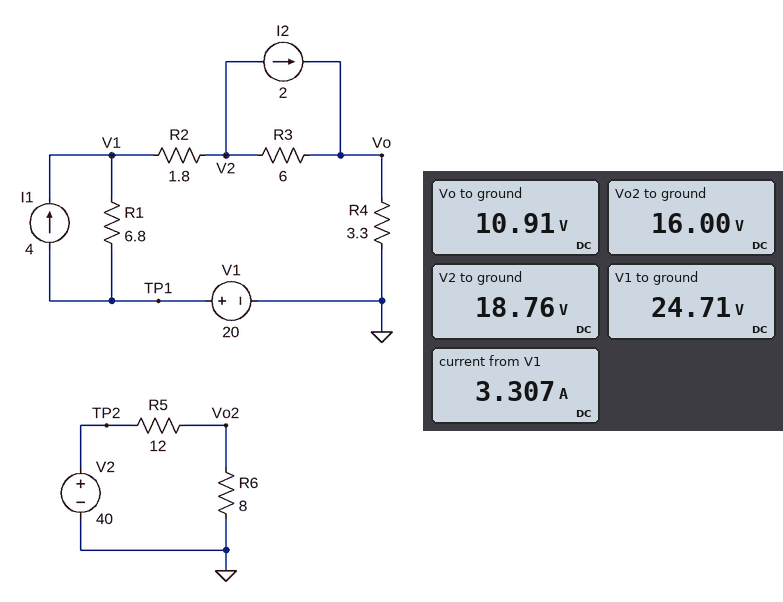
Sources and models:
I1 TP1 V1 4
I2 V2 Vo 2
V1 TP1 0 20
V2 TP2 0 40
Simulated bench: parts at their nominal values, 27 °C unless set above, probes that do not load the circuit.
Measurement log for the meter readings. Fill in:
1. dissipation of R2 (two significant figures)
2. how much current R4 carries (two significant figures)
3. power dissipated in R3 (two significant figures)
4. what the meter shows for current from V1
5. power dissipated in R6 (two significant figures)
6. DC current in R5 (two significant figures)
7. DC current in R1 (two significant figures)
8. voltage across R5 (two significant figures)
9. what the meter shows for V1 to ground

20 W
3.3 A
10 W
3.307 A
32 W
2.0 A
690 mA
24 V
24.71 V
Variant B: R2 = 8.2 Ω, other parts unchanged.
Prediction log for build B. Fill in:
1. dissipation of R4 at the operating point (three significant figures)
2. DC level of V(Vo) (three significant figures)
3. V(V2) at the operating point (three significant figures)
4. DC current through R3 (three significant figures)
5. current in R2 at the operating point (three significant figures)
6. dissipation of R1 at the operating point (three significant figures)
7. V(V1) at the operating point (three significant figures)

19.6 W
8.04 V
10.7 V
436 mA
2.44 A
16.6 W
30.6 V
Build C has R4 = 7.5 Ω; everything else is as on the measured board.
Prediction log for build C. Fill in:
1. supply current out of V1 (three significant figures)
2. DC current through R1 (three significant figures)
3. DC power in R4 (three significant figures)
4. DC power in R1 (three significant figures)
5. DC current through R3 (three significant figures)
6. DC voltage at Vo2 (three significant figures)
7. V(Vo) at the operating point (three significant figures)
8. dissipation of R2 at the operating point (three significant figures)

2.68 A
1.32 A
53.8 W
11.9 W
679 mA
16.0 V
20.1 V
12.9 W
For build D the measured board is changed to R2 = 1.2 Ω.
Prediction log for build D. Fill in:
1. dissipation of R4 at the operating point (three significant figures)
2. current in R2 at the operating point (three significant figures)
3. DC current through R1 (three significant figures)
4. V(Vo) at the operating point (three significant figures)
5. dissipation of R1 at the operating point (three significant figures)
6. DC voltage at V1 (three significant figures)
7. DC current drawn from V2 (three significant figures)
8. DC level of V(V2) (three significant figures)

38.6 W
3.42 A
578 mA
11.3 V
2.27 W
23.9 V
2.00 A
19.8 V
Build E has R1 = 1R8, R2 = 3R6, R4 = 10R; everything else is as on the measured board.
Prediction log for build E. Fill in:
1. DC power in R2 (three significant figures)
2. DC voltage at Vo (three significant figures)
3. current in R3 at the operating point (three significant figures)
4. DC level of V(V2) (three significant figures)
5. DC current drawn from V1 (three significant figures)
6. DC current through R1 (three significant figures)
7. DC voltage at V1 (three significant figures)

12.1 W
18.3 V
168 mA
17.3 V
1.83 A
2.17 A
23.9 V
